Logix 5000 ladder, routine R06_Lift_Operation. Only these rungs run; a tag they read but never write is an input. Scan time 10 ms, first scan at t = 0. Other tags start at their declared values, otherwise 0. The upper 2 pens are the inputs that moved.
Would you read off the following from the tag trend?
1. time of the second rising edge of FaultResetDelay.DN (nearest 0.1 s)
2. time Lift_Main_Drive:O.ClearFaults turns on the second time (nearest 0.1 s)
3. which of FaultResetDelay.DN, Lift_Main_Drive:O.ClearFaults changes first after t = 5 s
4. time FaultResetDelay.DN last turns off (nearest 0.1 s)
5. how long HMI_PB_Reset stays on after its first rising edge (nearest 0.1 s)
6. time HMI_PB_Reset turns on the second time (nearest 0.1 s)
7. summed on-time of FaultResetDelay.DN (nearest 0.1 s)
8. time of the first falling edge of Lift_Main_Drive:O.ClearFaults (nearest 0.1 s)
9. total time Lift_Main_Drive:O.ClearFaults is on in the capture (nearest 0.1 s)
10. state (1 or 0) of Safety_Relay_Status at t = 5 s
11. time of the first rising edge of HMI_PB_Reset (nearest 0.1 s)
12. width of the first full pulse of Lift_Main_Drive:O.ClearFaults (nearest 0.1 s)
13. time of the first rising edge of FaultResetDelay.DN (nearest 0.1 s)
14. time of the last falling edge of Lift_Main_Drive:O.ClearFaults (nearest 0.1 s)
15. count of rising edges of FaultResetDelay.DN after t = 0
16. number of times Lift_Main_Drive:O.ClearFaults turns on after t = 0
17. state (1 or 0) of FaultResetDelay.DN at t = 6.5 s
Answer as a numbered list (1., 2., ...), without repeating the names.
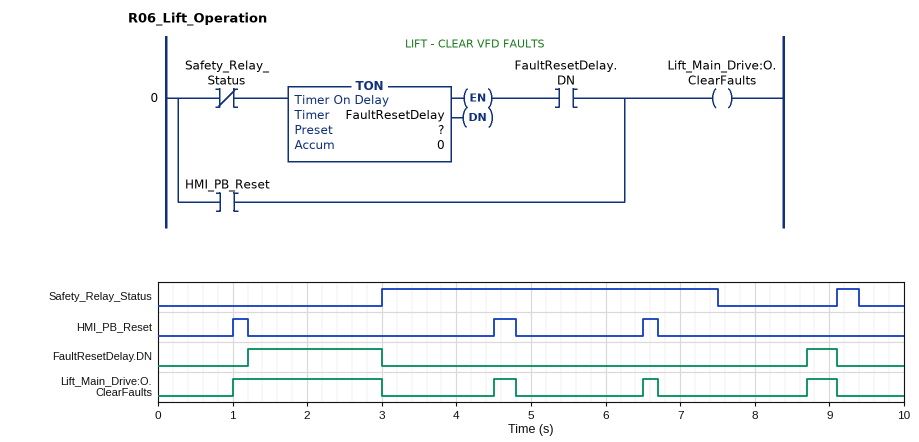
1. 8.7 s
2. 4.5 s
3. Lift_Main_Drive:O.ClearFaults
4. 9.1 s
5. 0.2 s
6. 4.5 s
7. 2.2 s
8. 3.0 s
9. 2.9 s
10. 1
11. 1.0 s
12. 2.0 s
13. 1.2 s
14. 9.1 s
15. 2
16. 4
17. 0
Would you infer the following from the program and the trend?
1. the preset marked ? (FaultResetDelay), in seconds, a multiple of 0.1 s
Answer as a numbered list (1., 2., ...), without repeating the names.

1. 1.2 s
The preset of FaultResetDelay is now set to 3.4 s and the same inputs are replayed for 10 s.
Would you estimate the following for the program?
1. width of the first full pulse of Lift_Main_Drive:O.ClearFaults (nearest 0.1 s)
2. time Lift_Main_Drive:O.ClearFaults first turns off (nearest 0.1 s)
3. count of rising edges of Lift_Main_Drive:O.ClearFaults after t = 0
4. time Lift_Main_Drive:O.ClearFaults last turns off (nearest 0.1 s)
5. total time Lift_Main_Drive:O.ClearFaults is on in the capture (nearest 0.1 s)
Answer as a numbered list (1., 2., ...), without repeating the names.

1. 0.2 s
2. 1.2 s
3. 3
4. 6.7 s
5. 0.7 s
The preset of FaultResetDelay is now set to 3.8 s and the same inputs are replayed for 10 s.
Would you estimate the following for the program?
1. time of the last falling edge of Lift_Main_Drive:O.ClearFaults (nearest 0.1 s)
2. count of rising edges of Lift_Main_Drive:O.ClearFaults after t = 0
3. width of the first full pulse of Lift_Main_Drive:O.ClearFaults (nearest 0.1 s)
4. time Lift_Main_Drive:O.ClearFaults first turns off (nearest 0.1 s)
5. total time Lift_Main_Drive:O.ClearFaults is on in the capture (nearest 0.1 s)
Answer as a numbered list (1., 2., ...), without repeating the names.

1. 6.7 s
2. 3
3. 0.2 s
4. 1.2 s
5. 0.7 s
